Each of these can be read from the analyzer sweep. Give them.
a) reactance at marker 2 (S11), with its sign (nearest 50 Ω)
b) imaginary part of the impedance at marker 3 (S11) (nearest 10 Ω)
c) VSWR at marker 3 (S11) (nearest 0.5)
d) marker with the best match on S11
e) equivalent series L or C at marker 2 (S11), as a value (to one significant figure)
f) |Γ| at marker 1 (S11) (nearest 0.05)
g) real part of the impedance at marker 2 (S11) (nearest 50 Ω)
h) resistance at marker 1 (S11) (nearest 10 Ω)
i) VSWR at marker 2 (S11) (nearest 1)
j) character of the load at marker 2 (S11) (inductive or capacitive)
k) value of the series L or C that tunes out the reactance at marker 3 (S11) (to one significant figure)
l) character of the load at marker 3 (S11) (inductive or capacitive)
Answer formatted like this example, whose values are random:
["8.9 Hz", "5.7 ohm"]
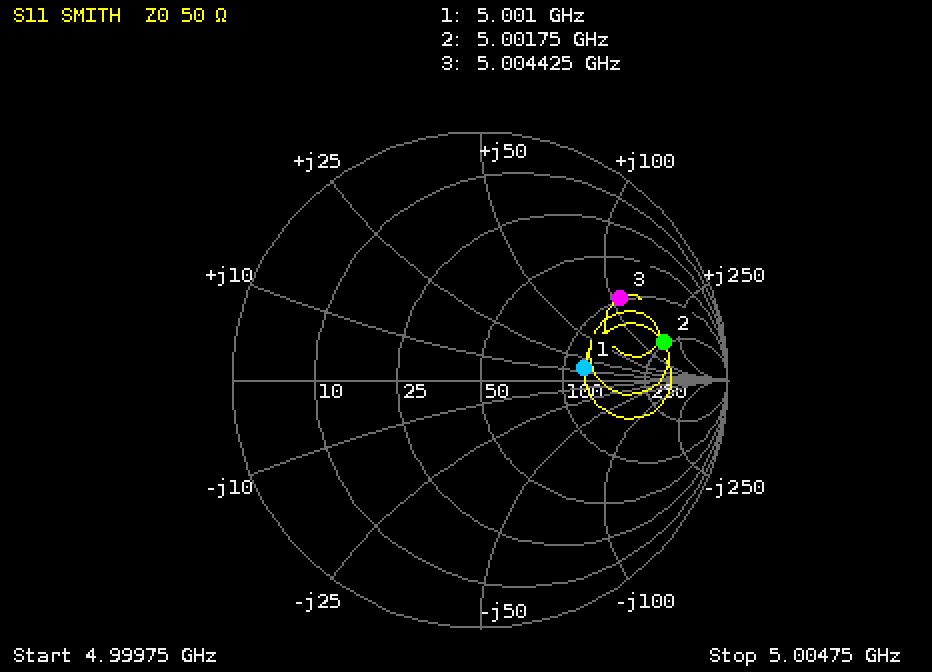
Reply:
["+150 Ω", "+110 Ω", "5.0", "marker 1", "5 nH", "0.40", "250 Ω", "120 Ω", "7", "inductive", "300 fF", "inductive"]
